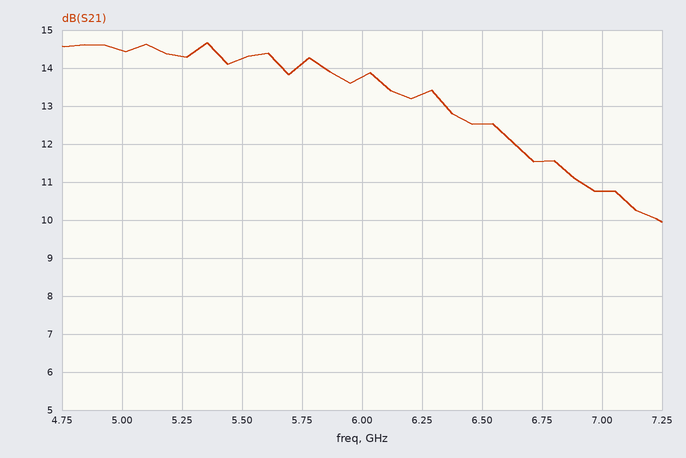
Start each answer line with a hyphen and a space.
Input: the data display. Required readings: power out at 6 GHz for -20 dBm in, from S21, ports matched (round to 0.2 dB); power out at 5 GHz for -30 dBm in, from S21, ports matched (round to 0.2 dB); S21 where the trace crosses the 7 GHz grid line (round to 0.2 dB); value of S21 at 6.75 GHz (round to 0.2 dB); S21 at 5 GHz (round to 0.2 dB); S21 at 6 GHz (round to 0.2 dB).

- -6.2 dBm
- -15.6 dBm
- 10.8 dB
- 11.6 dB
- 14.4 dB
- 13.8 dB
